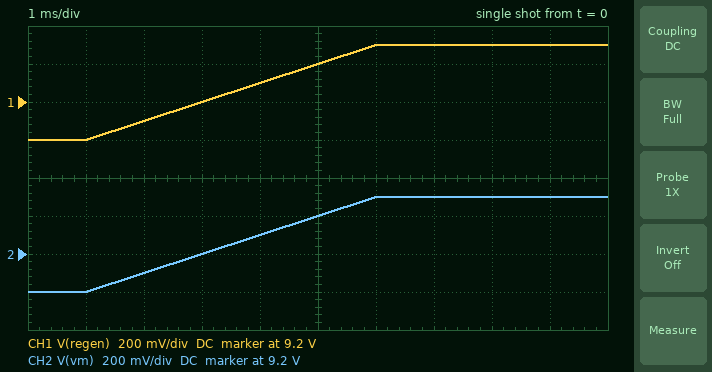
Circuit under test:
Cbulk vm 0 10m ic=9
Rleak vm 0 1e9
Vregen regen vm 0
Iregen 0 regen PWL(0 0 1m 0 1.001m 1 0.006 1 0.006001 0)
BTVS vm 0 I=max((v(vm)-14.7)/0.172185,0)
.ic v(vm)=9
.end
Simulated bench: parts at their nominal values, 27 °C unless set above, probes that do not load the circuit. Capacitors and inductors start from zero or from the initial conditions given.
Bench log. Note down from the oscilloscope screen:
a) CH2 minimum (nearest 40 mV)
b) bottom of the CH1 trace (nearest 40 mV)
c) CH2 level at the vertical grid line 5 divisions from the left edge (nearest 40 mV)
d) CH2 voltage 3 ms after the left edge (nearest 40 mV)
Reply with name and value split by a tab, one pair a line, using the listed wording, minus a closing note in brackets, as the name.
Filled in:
CH2 minimum	9.00 V
bottom of the CH1 trace	9.00 V
CH2 level at the vertical grid line 5 divisions from the left edge	9.40 V
CH2 voltage 3 ms after the left edge	9.20 V
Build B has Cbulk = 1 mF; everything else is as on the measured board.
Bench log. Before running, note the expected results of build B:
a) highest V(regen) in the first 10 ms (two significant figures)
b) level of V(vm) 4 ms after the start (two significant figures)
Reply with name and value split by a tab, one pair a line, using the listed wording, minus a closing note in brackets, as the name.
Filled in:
highest V(regen) in the first 10 ms	14 V
level of V(vm) 4 ms after the start	12 V
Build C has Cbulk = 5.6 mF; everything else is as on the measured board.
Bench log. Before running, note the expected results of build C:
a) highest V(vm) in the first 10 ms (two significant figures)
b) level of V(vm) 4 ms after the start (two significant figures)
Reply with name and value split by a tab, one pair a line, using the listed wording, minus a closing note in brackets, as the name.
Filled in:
highest V(vm) in the first 10 ms	9.9 V
level of V(vm) 4 ms after the start	9.5 V
